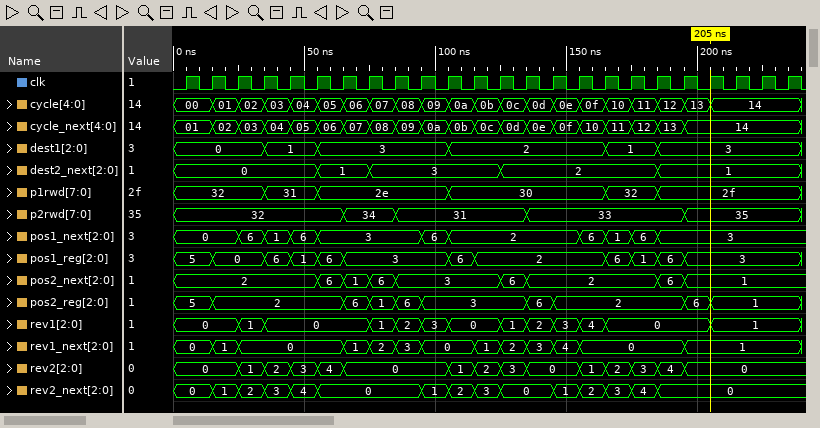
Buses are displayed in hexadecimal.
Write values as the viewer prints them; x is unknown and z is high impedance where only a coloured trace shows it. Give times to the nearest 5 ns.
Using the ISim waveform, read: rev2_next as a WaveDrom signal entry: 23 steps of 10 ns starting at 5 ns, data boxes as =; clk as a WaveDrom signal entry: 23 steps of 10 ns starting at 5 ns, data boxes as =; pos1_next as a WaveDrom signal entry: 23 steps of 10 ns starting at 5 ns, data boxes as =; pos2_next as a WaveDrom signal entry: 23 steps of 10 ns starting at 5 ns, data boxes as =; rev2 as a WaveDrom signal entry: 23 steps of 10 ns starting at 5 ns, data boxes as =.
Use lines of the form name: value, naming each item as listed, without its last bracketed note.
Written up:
rev2_next as a WaveDrom signal entry: 23 steps of 10 ns starting at 5 ns, data boxes as =: {name: 'rev2_next', wave: '======...====.=====....', data: '0 1 2 3 4 0 1 2 3 0 1 2 3 4 0'}
clk as a WaveDrom signal entry: 23 steps of 10 ns starting at 5 ns, data boxes as =: {name: 'clk', wave: 'p......................'}
pos1_next as a WaveDrom signal entry: 23 steps of 10 ns starting at 5 ns, data boxes as =: {name: 'pos1_next', wave: '=.====...==....====....', data: '0 6 1 6 3 6 2 6 1 6 3'}
pos2_next as a WaveDrom signal entry: 23 steps of 10 ns starting at 5 ns, data boxes as =: {name: 'pos2_next', wave: '=....====...==....==...', data: '2 6 1 6 3 6 2 6 1'}
rev2 as a WaveDrom signal entry: 23 steps of 10 ns starting at 5 ns, data boxes as =: {name: 'rev2', wave: '=.=====...====.=====...', data: '0 1 2 3 4 0 1 2 3 0 1 2 3 4 0'}
